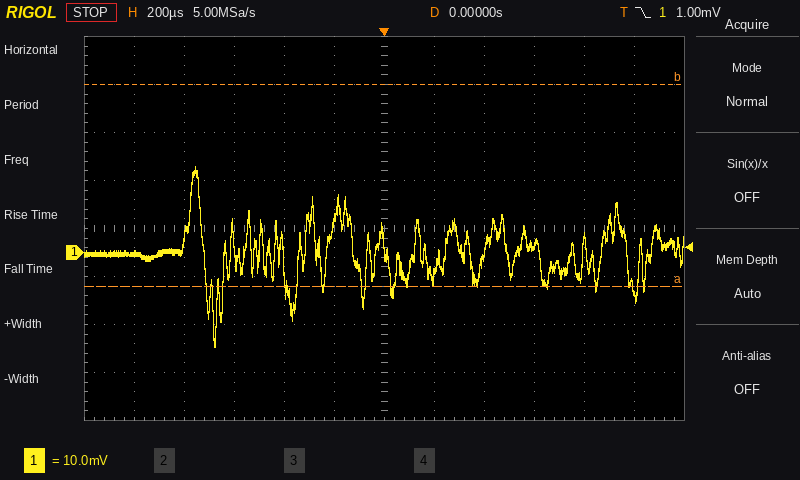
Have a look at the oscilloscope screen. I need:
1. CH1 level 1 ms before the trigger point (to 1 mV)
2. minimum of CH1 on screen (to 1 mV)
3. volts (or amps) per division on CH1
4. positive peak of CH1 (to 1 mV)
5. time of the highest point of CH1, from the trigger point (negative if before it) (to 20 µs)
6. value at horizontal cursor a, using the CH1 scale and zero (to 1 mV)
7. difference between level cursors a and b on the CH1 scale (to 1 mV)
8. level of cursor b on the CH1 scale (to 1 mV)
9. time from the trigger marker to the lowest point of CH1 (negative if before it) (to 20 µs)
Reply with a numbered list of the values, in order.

1. 0 mV
2. -20 mV
3. 10 mV
4. 18 mV
5. -760 µs
6. -7 mV
7. 42 mV
8. 35 mV
9. -680 µs
